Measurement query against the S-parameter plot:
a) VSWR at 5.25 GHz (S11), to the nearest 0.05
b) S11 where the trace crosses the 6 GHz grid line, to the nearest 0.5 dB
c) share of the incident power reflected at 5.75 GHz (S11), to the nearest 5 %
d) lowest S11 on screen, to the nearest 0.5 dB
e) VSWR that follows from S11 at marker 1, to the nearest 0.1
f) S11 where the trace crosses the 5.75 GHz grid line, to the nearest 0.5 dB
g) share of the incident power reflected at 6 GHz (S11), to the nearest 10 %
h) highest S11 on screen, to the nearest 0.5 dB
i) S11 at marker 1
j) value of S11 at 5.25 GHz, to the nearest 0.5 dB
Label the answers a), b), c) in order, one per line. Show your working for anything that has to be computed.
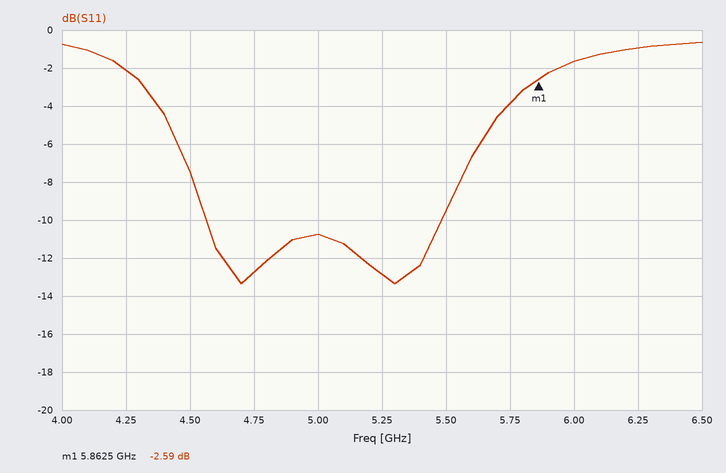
a) |Γ| = 10^(-13/20) = 0.2239; VSWR = (1 + 0.2239)/(1 − 0.2239) ≈ 1.58, so 1.60 to the nearest 0.05
b) -1.5 dB
c) 10^(-4/10) ≈ 40 %
d) -13.5 dB
e) (1 + 0.7422)/(1 − 0.7422) ≈ 6.8
f) -4.0 dB
g) 10^(-1.5/10) ≈ 70.8 %, so 70 % to the nearest 10 %
h) -0.5 dB
i) -2.59 dB
j) -13.0 dB
